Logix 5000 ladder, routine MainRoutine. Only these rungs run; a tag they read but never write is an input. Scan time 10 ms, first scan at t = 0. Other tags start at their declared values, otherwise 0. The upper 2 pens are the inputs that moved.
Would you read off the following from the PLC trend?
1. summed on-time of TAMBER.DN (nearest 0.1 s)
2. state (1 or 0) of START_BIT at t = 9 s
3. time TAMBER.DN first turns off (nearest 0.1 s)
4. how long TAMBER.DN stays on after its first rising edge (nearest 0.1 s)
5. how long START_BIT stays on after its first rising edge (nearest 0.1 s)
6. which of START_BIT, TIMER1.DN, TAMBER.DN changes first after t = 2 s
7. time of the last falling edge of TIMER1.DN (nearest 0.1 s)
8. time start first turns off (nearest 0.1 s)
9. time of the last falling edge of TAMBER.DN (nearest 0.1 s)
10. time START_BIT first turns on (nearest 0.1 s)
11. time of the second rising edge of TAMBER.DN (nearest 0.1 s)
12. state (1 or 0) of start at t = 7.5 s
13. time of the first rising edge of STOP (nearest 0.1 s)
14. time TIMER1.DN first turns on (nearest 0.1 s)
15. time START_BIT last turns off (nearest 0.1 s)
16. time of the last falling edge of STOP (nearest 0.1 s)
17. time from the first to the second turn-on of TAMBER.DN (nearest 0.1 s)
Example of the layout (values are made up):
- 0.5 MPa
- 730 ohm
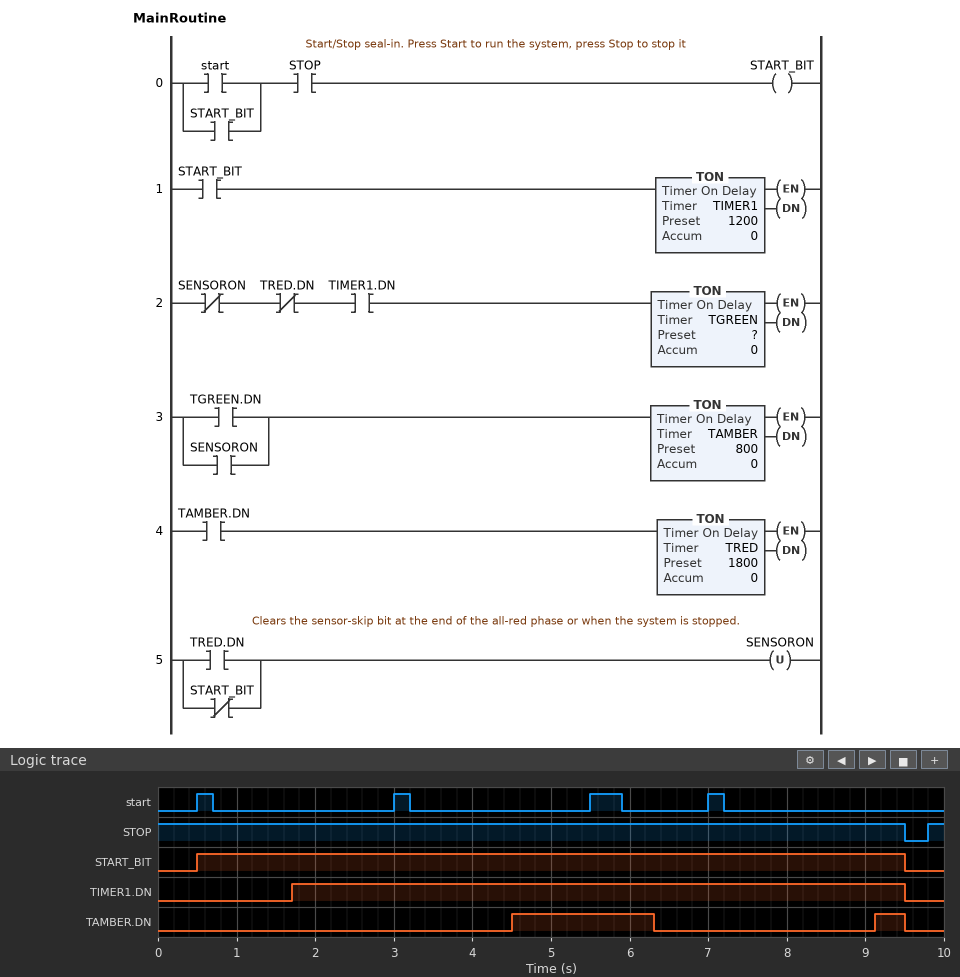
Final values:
- 2.2 s
- 1
- 6.3 s
- 1.8 s
- 9.0 s
- TAMBER.DN
- 9.5 s
- 0.7 s
- 9.5 s
- 0.5 s
- 9.1 s
- 0
- 9.8 s
- 1.7 s
- 9.5 s
- 9.5 s
- 4.6 s
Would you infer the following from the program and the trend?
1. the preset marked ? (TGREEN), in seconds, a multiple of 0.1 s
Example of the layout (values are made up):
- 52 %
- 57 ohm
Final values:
- 2.0 s
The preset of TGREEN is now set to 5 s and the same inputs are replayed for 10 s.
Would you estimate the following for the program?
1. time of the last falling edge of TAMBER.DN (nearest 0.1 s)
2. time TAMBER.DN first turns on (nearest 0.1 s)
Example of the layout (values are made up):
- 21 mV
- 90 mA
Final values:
- 9.3 s
- 7.5 s
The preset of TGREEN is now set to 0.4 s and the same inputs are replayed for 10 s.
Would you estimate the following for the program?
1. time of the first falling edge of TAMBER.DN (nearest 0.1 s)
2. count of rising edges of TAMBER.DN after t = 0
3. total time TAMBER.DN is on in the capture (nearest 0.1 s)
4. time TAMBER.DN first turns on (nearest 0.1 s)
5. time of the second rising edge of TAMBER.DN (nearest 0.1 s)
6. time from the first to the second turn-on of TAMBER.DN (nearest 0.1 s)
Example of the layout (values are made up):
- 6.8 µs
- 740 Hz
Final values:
- 4.7 s
- 3
- 4.2 s
- 2.9 s
- 5.9 s
- 3.0 s
